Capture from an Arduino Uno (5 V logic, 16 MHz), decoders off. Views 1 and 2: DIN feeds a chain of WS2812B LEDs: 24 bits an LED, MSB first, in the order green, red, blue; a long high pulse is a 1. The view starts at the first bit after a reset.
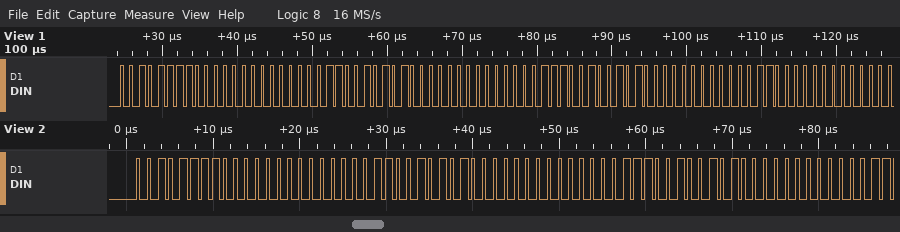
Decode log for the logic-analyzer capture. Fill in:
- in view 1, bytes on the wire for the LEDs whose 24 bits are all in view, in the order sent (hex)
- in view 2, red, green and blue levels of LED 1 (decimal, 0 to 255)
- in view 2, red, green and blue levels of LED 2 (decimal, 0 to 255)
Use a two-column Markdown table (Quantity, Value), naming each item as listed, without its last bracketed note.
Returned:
| Quantity | Value |
|---|---|
| in view 1, bytes on the wire for the LEDs whose 24 bits are all in view, in the order sent | 2F 00 03 2A 00 07 25 00 0C |
| in view 2, red, green and blue levels of LED 1 | 0, 47, 3 |
| in view 2, red, green and blue levels of LED 2 | 0, 42, 7 |
